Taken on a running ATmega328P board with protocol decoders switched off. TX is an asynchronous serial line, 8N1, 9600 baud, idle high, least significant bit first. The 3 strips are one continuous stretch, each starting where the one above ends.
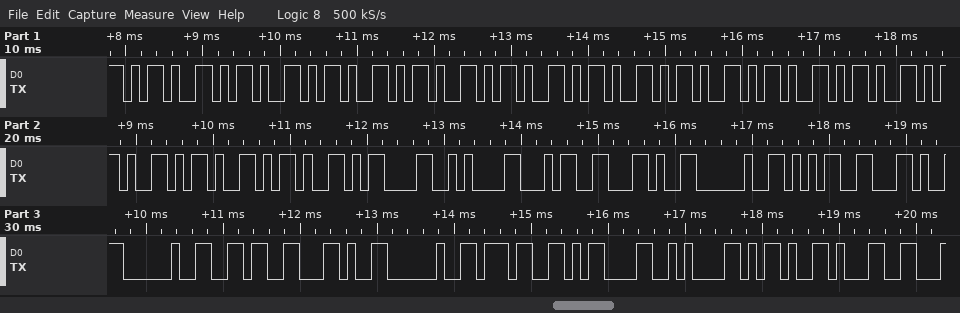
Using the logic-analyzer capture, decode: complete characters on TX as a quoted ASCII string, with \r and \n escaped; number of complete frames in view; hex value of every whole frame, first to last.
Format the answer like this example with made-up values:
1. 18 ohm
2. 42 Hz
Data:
1. "------------\r\n4, 5, 6, 7\r\n-1"
2. 28
3. 0x2D 0x2D 0x2D 0x2D 0x2D 0x2D 0x2D 0x2D 0x2D 0x2D 0x2D 0x2D 0x0D 0x0A 0x34 0x2C 0x20 0x35 0x2C 0x20 0x36 0x2C 0x20 0x37 0x0D 0x0A 0x2D 0x31
